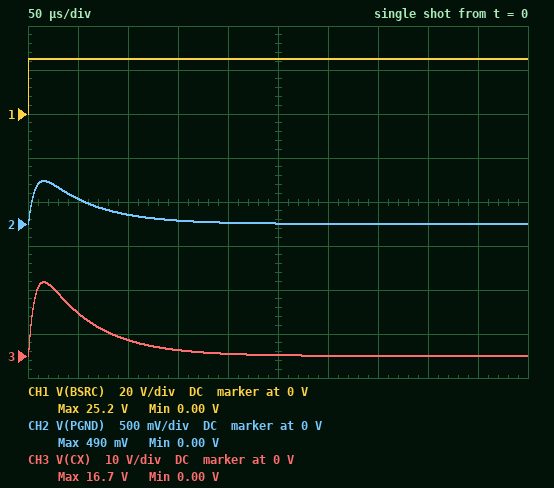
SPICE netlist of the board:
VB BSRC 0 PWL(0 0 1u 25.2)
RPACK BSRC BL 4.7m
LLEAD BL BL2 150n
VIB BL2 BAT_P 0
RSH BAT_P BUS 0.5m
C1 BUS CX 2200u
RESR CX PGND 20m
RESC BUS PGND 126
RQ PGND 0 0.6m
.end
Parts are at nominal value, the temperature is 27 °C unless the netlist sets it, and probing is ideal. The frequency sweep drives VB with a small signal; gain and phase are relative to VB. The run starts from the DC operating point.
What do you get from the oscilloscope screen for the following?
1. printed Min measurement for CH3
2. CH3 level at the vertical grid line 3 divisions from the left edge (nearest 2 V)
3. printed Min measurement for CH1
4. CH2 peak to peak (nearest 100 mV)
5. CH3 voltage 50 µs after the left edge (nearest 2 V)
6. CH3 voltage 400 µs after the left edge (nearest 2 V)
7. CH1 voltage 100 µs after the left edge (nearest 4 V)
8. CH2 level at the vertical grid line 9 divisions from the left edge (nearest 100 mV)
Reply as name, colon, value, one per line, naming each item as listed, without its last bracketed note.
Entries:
printed Min measurement for CH3: 0.00 V
CH3 level at the vertical grid line 3 divisions from the left edge: 2 V
printed Min measurement for CH1: 0.00 V
CH2 peak to peak: 500 mV
CH3 voltage 50 µs after the left edge: 10 V
CH3 voltage 400 µs after the left edge: 0 V
CH1 voltage 100 µs after the left edge: 24 V
CH2 level at the vertical grid line 9 divisions from the left edge: 0 V
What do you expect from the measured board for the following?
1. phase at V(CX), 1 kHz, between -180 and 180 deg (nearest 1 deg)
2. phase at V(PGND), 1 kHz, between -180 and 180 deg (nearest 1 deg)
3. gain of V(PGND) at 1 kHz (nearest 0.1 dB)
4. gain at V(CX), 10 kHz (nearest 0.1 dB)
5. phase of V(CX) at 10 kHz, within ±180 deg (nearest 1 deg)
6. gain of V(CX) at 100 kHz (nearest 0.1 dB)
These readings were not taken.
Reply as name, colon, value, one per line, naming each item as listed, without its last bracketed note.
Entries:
phase at V(CX), 1 kHz, between -180 and 180 deg: 70 deg
phase at V(PGND), 1 kHz, between -180 and 180 deg: 70 deg
gain of V(PGND) at 1 kHz: -42.0 dB
gain at V(CX), 10 kHz: -2.0 dB
phase of V(CX) at 10 kHz, within ±180 deg: -5 deg
gain of V(CX) at 100 kHz: -13.5 dB
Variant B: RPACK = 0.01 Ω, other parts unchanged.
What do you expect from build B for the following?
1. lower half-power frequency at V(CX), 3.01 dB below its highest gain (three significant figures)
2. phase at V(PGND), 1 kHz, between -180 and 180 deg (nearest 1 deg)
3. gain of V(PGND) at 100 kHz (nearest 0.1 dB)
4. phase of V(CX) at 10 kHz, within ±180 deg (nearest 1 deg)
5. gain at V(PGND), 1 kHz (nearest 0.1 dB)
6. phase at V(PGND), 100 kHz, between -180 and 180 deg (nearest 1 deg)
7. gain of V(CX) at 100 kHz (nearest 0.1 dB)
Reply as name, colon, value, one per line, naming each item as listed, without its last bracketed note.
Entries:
lower half-power frequency at V(CX), 3.01 dB below its highest gain: 2.18 kHz
phase at V(PGND), 1 kHz, between -180 and 180 deg: 66 deg
gain of V(PGND) at 100 kHz: -44.3 dB
phase of V(CX) at 10 kHz, within ±180 deg: -4 deg
gain at V(PGND), 1 kHz: -42.3 dB
phase at V(PGND), 100 kHz, between -180 and 180 deg: -72 deg
gain of V(CX) at 100 kHz: -13.6 dB
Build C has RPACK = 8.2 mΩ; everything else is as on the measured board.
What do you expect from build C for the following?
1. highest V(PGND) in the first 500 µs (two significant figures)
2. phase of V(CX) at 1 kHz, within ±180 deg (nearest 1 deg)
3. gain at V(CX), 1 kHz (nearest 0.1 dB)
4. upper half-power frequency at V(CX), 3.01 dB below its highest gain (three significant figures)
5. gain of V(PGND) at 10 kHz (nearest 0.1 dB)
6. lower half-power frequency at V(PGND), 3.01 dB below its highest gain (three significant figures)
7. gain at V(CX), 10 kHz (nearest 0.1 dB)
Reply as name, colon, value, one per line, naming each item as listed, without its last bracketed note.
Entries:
highest V(PGND) in the first 500 µs: 440 mV
phase of V(CX) at 1 kHz, within ±180 deg: 68 deg
gain at V(CX), 1 kHz: -11.5 dB
upper half-power frequency at V(CX), 3.01 dB below its highest gain: 33.4 kHz
gain of V(PGND) at 10 kHz: -33.8 dB
lower half-power frequency at V(PGND), 3.01 dB below its highest gain: 2.30 kHz
gain at V(CX), 10 kHz: -3.1 dB
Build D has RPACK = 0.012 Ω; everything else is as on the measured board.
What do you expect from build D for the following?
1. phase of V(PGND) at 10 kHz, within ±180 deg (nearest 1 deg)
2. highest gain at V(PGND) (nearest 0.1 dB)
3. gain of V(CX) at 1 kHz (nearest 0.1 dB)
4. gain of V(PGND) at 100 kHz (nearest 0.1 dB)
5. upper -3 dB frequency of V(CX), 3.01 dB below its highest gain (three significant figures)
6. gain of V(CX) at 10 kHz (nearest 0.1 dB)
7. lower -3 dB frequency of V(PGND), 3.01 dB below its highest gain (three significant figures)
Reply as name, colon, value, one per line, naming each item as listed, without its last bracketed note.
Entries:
phase of V(PGND) at 10 kHz, within ±180 deg: -4 deg
highest gain at V(PGND): -34.8 dB
gain of V(CX) at 1 kHz: -11.6 dB
gain of V(PGND) at 100 kHz: -44.4 dB
upper -3 dB frequency of V(CX), 3.01 dB below its highest gain: 37.2 kHz
gain of V(CX) at 10 kHz: -4.1 dB
lower -3 dB frequency of V(PGND), 3.01 dB below its highest gain: 2.06 kHz
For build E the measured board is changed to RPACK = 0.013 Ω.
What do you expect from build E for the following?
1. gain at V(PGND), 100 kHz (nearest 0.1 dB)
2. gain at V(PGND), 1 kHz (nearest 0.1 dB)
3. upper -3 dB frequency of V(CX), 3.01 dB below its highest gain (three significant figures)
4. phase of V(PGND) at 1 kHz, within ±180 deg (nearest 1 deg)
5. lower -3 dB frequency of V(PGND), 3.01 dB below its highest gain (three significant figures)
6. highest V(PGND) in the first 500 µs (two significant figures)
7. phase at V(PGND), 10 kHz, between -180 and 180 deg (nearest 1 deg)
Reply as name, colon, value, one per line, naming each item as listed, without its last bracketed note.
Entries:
gain at V(PGND), 100 kHz: -44.4 dB
gain at V(PGND), 1 kHz: -42.4 dB
upper -3 dB frequency of V(CX), 3.01 dB below its highest gain: 38.2 kHz
phase of V(PGND) at 1 kHz, within ±180 deg: 64 deg
lower -3 dB frequency of V(PGND), 3.01 dB below its highest gain: 2.01 kHz
highest V(PGND) in the first 500 µs: 390 mV
phase at V(PGND), 10 kHz, between -180 and 180 deg: -4 deg
